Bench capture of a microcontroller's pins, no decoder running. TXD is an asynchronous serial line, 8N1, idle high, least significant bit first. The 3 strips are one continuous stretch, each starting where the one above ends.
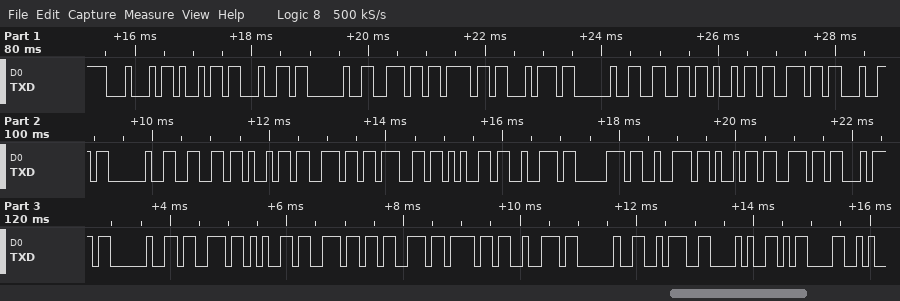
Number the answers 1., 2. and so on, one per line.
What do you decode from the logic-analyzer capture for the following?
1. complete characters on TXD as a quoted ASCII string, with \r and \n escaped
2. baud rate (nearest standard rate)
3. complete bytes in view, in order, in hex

1. "Did not find fingerprint sensor :(\r"
2. 9600 baud
3. 44 69 64 20 6E 6F 74 20 66 69 6E 64 20 66 69 6E 67 65 72 70 72 69 6E 74 20 73 65 6E 73 6F 72 20 3A 28 0D
